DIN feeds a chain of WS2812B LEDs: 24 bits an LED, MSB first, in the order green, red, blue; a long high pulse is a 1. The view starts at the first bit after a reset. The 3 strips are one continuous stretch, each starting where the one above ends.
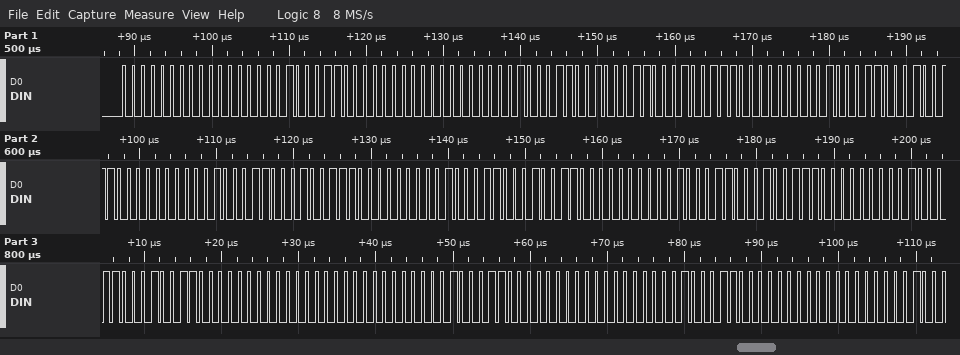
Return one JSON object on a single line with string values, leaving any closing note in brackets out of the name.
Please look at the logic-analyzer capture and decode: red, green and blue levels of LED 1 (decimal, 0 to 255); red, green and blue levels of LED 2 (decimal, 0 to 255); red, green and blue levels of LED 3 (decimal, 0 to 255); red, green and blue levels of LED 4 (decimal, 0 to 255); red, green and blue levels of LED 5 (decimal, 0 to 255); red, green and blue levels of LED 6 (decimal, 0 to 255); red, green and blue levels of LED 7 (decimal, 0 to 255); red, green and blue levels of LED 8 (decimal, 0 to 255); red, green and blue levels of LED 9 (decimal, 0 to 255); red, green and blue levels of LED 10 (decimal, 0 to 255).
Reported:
{"red, green and blue levels of LED 1": "0, 0, 70", "red, green and blue levels of LED 2": "0, 0, 70", "red, green and blue levels of LED 3": "39, 70, 0", "red, green and blue levels of LED 4": "38, 70, 0", "red, green and blue levels of LED 5": "39, 70, 0", "red, green and blue levels of LED 6": "38, 70, 0", "red, green and blue levels of LED 7": "39, 70, 0", "red, green and blue levels of LED 8": "38, 70, 0", "red, green and blue levels of LED 9": "0, 0, 70", "red, green and blue levels of LED 10": "0, 0, 70"}
